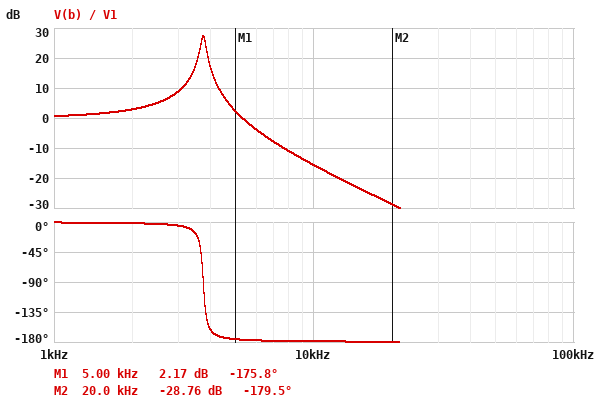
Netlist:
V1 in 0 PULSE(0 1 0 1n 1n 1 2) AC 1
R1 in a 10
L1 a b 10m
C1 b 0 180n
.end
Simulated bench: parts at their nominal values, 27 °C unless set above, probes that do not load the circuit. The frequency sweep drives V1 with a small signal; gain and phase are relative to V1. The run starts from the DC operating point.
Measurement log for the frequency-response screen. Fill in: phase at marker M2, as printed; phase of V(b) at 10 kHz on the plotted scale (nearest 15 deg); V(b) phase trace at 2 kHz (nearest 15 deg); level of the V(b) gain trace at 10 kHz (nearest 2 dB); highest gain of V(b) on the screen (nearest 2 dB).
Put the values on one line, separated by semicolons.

-179.5 deg; -180 deg; 0 deg; -16 dB; 28 dB
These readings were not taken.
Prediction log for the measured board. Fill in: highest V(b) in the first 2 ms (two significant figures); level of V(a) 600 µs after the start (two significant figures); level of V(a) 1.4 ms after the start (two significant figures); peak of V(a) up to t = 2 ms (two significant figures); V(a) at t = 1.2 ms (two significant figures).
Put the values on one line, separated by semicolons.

1.9 V; 970 mV; 980 mV; 1.0 V; 1.0 V
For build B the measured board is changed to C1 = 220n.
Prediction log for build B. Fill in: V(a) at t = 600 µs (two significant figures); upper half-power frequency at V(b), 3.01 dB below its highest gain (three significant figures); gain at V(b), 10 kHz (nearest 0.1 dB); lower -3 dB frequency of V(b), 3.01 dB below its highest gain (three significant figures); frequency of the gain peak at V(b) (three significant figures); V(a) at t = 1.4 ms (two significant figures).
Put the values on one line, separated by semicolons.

990 mV; 3.47 kHz; -17.7 dB; 3.31 kHz; 3.39 kHz; 1.0 V
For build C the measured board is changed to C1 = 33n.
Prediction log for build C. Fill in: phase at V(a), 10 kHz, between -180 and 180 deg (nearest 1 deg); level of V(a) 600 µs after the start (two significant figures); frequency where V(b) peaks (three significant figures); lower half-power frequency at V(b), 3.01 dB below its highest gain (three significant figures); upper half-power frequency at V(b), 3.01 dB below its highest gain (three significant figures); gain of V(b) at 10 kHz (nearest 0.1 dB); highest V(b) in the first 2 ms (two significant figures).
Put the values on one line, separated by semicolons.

4 deg; 990 mV; 8.76 kHz; 8.68 kHz; 8.84 kHz; 10.4 dB; 2.0 V
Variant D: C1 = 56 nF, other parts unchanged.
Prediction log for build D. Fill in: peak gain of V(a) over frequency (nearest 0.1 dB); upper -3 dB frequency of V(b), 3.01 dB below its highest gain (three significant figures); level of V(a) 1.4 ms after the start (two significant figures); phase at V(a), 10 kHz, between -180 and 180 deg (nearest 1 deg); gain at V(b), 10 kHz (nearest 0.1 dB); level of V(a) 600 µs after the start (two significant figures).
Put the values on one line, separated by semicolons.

0 dB; 6.80 kHz; 990 mV; 2 deg; -1.7 dB; 1.0 V
